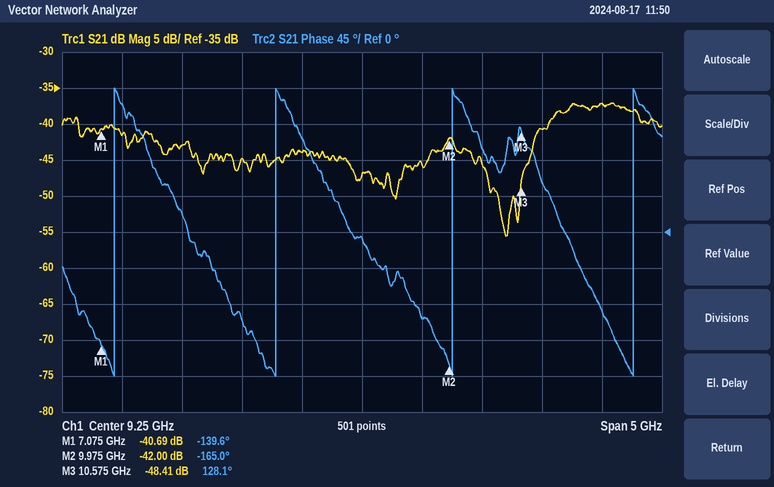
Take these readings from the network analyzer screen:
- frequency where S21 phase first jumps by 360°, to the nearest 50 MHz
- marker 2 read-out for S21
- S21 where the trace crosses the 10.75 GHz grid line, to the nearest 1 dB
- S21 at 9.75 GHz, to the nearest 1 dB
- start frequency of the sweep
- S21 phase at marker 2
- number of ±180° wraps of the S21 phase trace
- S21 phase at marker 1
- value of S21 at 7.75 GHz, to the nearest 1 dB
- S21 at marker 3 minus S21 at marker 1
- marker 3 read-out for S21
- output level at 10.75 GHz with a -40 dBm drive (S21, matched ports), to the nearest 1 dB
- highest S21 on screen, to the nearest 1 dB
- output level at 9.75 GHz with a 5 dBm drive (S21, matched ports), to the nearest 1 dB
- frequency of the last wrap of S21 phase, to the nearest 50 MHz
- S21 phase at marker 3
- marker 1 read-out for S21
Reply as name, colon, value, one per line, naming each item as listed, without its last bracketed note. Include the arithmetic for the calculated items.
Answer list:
frequency where S21 phase first jumps by 360°, to the nearest 50 MHz: 7.20 GHz
marker 2 read-out for S21: -42.00 dB
S21 where the trace crosses the 10.75 GHz grid line, to the nearest 1 dB: -41 dB
S21 at 9.75 GHz, to the nearest 1 dB: -46 dB
start frequency of the sweep: 6.75 GHz
S21 phase at marker 2: -165.0°
number of ±180° wraps of the S21 phase trace: 4
S21 phase at marker 1: -139.6°
value of S21 at 7.75 GHz, to the nearest 1 dB: -43 dB
S21 at marker 3 minus S21 at marker 1: -48.41 − (-40.69) = -7.72 dB
marker 3 read-out for S21: -48.41 dB
output level at 10.75 GHz with a -40 dBm drive (S21, matched ports), to the nearest 1 dB: -40 dBm + (-41 dB) = -81 dBm
highest S21 on screen, to the nearest 1 dB: -37 dB
output level at 9.75 GHz with a 5 dBm drive (S21, matched ports), to the nearest 1 dB: 5 dBm + (-46 dB) = -41 dBm
frequency of the last wrap of S21 phase, to the nearest 50 MHz: 11.50 GHz
S21 phase at marker 3: 128.1°
marker 1 read-out for S21: -40.69 dB
